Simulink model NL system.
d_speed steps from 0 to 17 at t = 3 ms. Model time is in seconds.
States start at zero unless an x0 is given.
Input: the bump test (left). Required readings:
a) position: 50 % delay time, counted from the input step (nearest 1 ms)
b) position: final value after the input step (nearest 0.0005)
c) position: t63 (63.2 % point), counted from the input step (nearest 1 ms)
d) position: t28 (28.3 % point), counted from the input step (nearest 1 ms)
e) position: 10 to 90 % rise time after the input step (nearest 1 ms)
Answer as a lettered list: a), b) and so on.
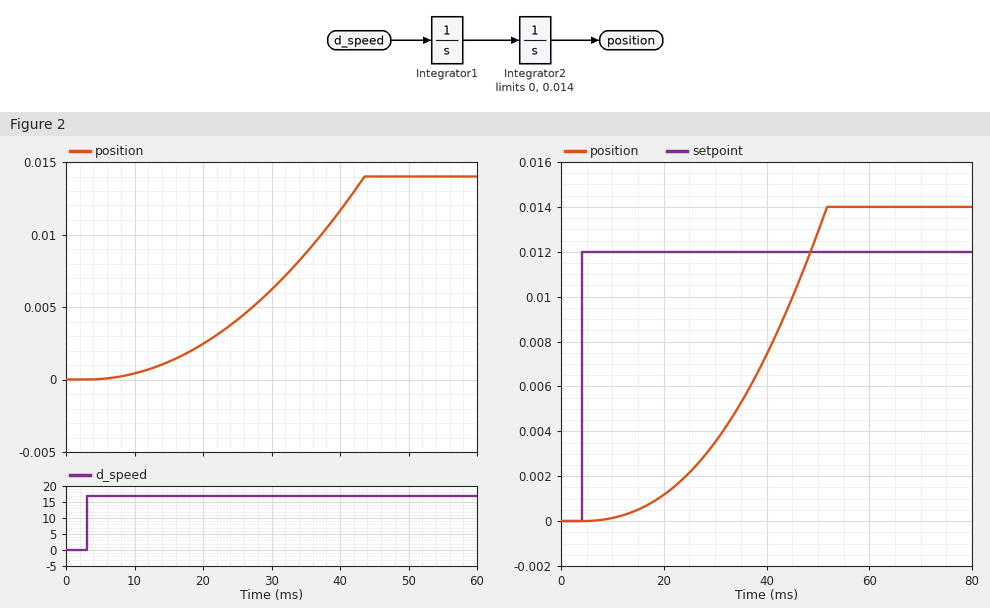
a) 29 ms
b) 0.0140
c) 32 ms
d) 22 ms
e) 26 ms
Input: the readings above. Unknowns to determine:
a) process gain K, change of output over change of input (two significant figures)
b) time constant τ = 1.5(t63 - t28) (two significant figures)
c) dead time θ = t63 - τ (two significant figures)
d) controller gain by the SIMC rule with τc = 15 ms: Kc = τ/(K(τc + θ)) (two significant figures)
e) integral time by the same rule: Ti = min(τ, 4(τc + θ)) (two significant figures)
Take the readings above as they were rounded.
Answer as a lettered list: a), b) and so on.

a) 0.00082
b) 15 ms
c) 17 ms
d) 570
e) 15 ms
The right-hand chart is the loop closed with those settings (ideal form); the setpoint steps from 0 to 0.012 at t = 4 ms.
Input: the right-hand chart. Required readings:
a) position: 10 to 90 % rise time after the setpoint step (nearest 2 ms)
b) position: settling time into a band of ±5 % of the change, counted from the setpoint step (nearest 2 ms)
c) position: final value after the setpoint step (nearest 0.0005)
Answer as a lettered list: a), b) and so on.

a) 28 ms
b) 46 ms
c) 0.0140
